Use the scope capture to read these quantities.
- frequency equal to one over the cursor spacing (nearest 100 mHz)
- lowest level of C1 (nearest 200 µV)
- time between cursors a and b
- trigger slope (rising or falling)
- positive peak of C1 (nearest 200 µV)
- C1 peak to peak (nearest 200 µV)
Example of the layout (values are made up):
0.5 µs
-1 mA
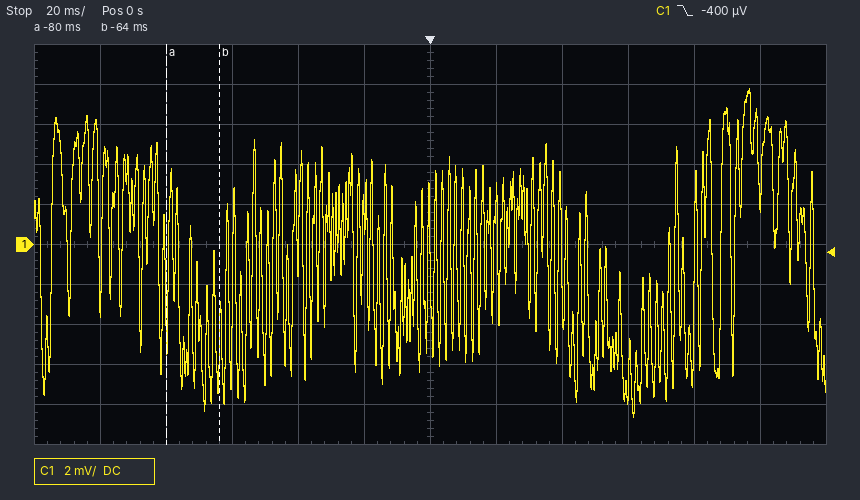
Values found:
62.5 Hz
-8.6 mV
16 ms
falling
7.8 mV
16.4 mV
